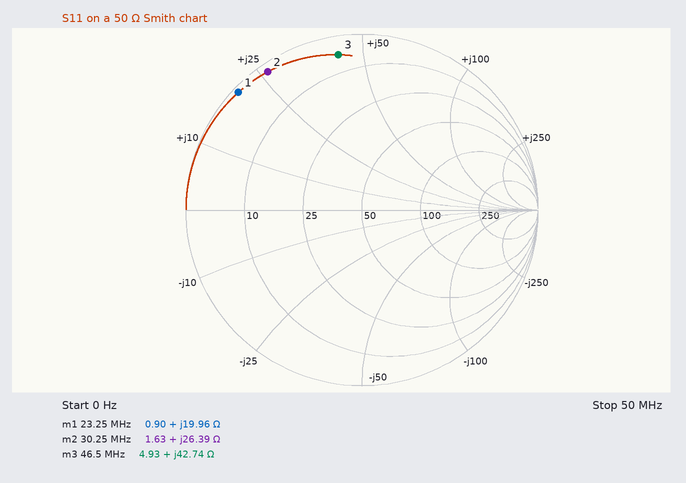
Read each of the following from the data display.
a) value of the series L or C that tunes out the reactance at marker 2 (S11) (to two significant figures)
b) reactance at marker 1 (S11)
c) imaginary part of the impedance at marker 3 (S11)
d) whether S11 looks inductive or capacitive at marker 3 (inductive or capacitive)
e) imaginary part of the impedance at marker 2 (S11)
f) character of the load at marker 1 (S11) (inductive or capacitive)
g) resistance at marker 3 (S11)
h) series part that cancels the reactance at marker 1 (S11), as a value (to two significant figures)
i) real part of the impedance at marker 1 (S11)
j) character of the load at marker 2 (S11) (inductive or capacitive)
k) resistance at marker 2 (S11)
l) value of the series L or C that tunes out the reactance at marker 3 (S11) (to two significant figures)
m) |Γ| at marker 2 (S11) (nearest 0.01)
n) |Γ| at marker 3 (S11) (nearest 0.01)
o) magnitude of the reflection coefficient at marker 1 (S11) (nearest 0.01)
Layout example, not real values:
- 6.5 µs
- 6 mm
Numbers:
- 200 pF
- +19.96 Ω
- +42.74 Ω
- inductive
- +26.39 Ω
- inductive
- 4.93 Ω
- 340 pF
- 0.90 Ω
- inductive
- 1.63 Ω
- 80 pF
- 0.95
- 0.89
- 0.97
